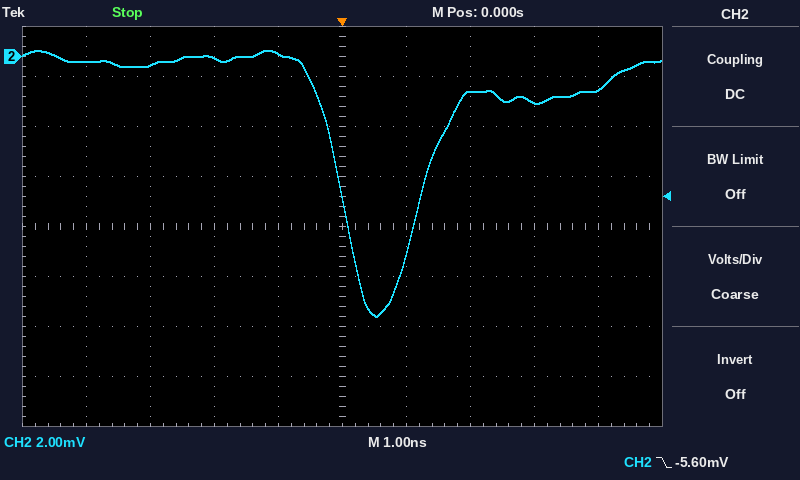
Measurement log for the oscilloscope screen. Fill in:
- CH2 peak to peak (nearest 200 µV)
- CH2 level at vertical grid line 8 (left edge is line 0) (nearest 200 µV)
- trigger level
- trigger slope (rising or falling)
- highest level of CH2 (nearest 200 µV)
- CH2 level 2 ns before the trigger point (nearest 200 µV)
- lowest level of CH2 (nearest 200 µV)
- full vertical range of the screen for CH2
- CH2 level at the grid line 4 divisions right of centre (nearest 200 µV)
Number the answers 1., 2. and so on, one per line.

1. 10.6 mV
2. -1.8 mV
3. -5.60 mV
4. falling
5. 200 µV
6. 0.0 mV
7. -10.4 mV
8. 16 mV
9. -1.4 mV
